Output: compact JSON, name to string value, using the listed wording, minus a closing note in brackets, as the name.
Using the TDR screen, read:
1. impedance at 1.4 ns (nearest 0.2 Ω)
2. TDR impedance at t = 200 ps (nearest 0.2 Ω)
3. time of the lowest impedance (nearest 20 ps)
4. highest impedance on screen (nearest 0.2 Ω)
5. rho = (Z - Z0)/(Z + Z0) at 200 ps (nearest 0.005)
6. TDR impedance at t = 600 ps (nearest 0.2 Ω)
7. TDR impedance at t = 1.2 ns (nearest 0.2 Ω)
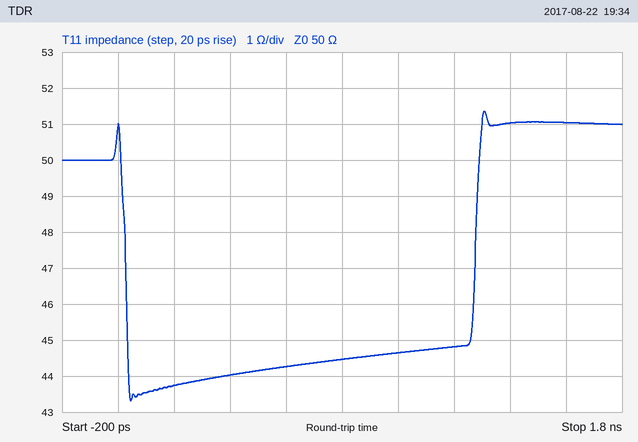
{"impedance at 1.4 ns": "51.0 Ω", "TDR impedance at t = 200 ps": "43.8 Ω", "time of the lowest impedance": "40 ps", "highest impedance on screen": "51.4 Ω", "rho = (Z - Z0)/(Z + Z0) at 200 ps": "-0.065", "TDR impedance at t = 600 ps": "44.2 Ω", "TDR impedance at t = 1.2 ns": "44.8 Ω"}
